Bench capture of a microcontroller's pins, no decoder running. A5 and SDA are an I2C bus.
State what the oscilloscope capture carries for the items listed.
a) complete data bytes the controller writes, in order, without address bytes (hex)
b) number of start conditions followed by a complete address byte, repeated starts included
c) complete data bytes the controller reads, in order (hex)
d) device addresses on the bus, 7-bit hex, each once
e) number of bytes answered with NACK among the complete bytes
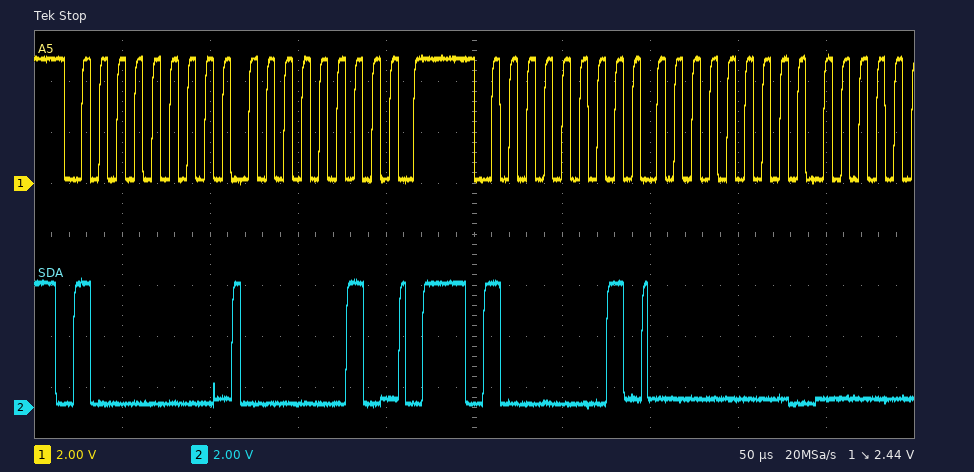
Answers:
02
2
00
0x40
0
